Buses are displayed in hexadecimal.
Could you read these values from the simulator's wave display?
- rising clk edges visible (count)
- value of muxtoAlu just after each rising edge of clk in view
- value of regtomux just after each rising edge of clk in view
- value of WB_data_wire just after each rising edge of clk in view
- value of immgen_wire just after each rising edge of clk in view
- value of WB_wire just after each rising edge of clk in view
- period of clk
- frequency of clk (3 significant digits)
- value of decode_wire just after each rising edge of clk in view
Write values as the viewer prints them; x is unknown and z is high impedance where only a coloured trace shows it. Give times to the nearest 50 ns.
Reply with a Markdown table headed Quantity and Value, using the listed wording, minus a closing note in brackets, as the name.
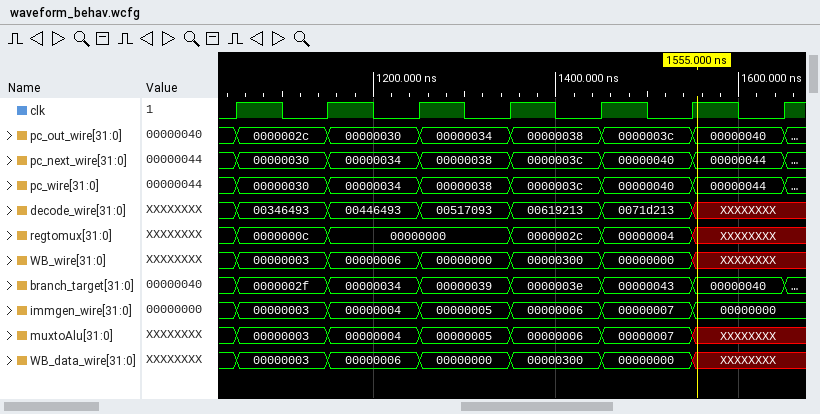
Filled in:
| Quantity | Value |
|---|---|
| rising clk edges visible | 7 |
| value of muxtoAlu just after each rising edge of clk in view | 00000003, 00000004, 00000005, 00000006, 00000007, XXXXXXXX, XXXXXXXX |
| value of regtomux just after each rising edge of clk in view | 0000000c, 00000000, 00000000, 0000002c, 00000004, XXXXXXXX, XXXXXXXX |
| value of WB_data_wire just after each rising edge of clk in view | 00000003, 00000006, 00000000, 00000300, 00000000, XXXXXXXX, XXXXXXXX |
| value of immgen_wire just after each rising edge of clk in view | 00000003, 00000004, 00000005, 00000006, 00000007, 00000000, 00000000 |
| value of WB_wire just after each rising edge of clk in view | 00000003, 00000006, 00000000, 00000300, 00000000, XXXXXXXX, XXXXXXXX |
| period of clk | 100 ns |
| frequency of clk | 10.0 MHz |
| value of decode_wire just after each rising edge of clk in view | 00346493, 00446493, 00517093, 00619213, 0071d213, XXXXXXXX, XXXXXXXX |
